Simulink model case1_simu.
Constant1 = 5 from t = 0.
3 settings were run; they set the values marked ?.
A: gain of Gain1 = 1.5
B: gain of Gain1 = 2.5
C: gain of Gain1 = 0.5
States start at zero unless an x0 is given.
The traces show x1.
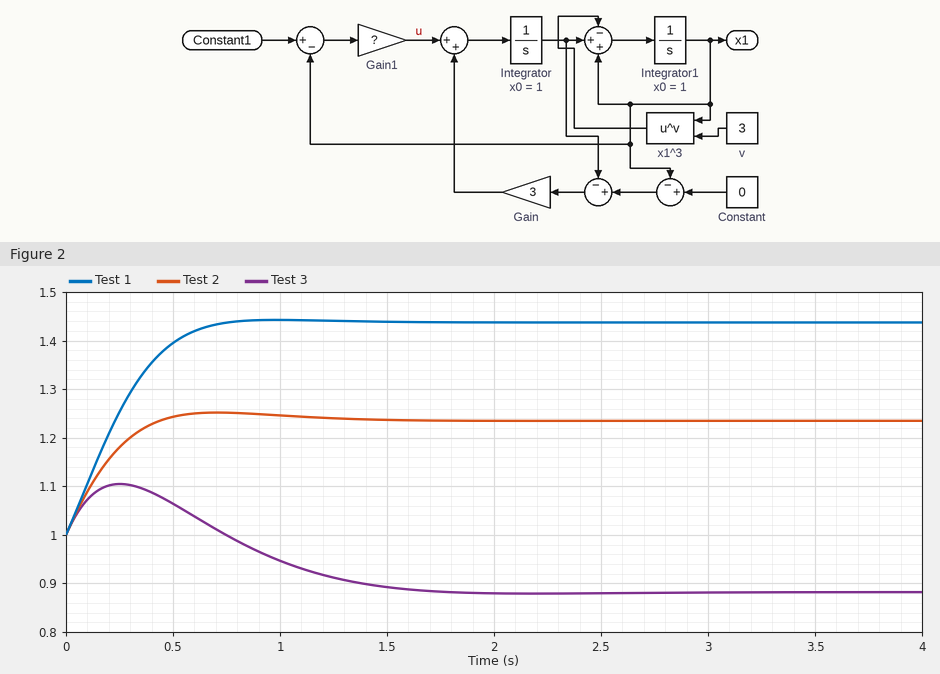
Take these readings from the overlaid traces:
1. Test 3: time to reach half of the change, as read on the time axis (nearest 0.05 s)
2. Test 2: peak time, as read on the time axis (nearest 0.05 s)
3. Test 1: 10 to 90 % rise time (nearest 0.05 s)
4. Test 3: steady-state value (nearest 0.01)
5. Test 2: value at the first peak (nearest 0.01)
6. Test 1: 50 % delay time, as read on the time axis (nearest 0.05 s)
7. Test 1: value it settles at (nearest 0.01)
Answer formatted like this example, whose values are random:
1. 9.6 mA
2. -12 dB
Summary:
1. 1.05 s
2. 0.70 s
3. 0.45 s
4. 0.88
5. 1.25
6. 0.20 s
7. 1.44
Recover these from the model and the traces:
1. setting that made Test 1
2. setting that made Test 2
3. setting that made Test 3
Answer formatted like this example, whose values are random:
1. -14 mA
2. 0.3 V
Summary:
1. B
2. A
3. C
